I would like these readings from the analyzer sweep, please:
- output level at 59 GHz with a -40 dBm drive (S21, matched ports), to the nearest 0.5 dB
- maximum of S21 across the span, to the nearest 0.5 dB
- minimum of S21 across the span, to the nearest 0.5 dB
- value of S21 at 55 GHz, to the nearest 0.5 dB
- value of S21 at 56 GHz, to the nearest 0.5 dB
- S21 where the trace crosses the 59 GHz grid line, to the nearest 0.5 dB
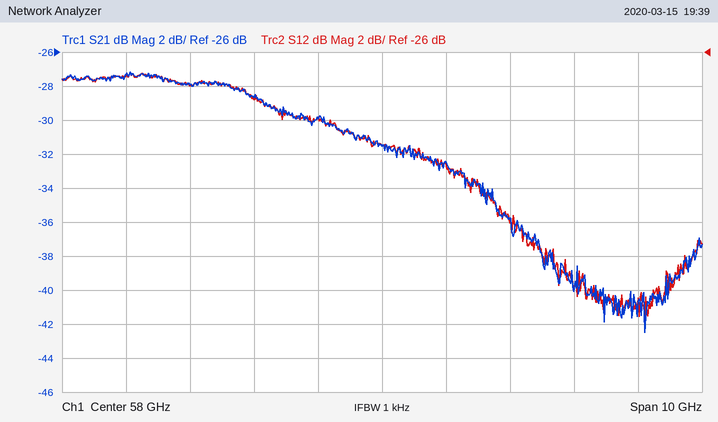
-72.5 dBm
-27.0 dB
-42.5 dB
-28.0 dB
-28.5 dB
-32.5 dB
